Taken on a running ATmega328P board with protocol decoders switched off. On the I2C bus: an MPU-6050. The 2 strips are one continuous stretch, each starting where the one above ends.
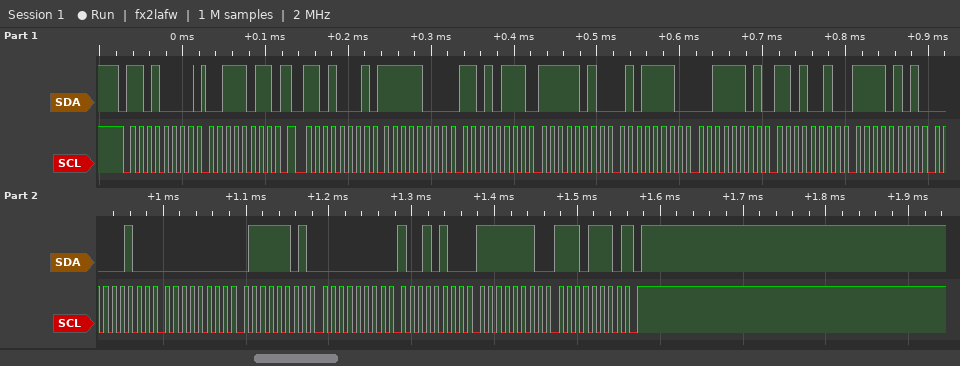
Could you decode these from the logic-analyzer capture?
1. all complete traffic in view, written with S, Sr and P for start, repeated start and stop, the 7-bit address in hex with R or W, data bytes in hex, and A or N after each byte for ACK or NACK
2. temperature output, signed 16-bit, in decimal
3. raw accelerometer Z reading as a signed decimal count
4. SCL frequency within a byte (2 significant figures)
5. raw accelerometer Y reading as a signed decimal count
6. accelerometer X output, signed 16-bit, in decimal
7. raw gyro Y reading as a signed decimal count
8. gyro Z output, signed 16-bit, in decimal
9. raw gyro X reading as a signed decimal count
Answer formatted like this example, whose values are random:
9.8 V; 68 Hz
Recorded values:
S 68W A 3B A Sr 68R A F8 A D7 A FA A 5E A 3D A D2 A F5 A 04 A 00 A 7D A 00 A 94 A FE A EE N P; -2812; 15826; 100 kHz; -1442; -1833; 148; -274; 125
